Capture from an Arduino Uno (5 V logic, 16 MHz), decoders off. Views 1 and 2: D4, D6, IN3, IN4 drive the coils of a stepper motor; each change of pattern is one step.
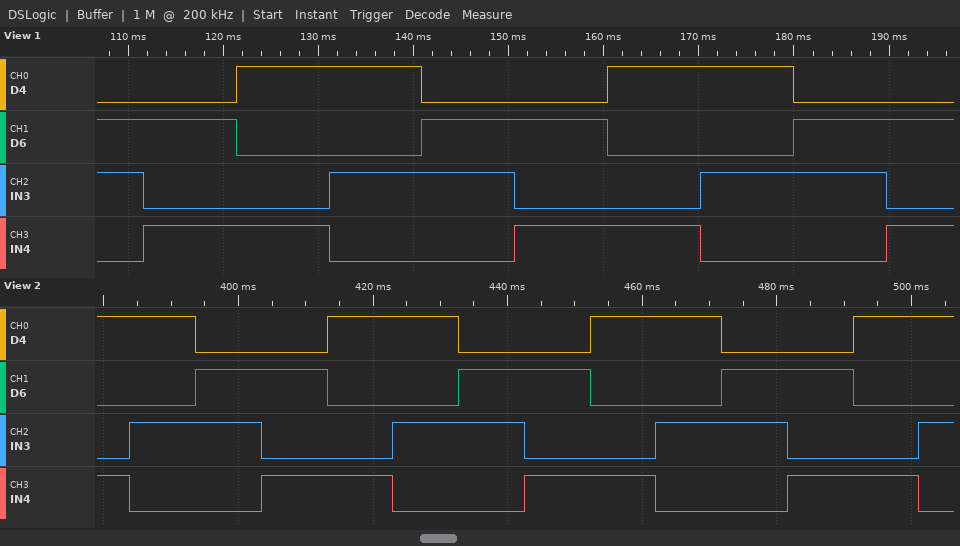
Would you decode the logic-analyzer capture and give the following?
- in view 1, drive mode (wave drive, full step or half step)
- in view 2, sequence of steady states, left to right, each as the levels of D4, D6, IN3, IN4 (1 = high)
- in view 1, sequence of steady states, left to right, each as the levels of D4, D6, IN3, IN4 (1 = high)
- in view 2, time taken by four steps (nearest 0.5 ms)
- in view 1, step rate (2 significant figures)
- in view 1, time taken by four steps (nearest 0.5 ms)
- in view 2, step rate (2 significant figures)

full step
1001 1010 0110 0101 1001 1010 0110 0101 1001 1010 0110 0101 1001 1010
0110 0101 1001 1010 0110 0101 1001 1010 0110 0101
39.0 ms
100 steps/s
39.0 ms
100 steps/s
